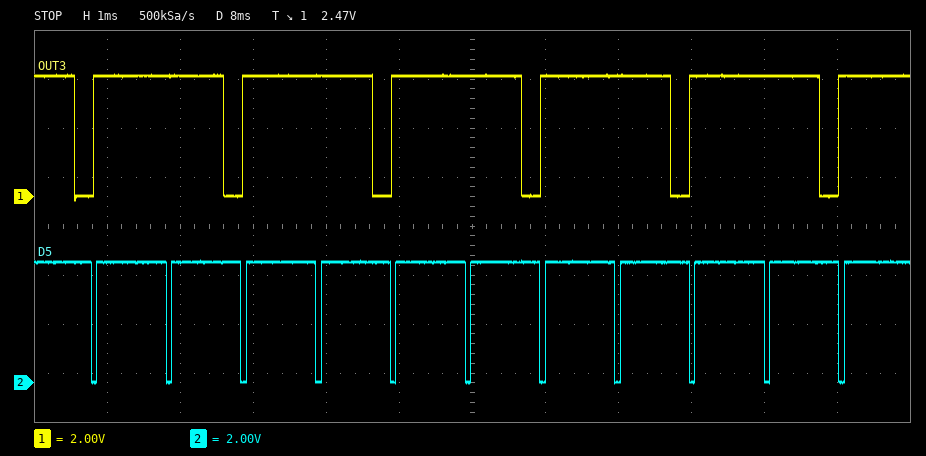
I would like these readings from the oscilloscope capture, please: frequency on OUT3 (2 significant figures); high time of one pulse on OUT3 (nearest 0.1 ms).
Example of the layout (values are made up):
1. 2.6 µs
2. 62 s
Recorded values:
1. 490 Hz
2. 1.8 ms
